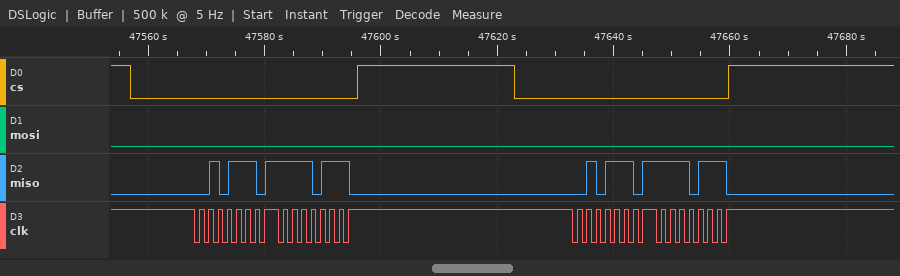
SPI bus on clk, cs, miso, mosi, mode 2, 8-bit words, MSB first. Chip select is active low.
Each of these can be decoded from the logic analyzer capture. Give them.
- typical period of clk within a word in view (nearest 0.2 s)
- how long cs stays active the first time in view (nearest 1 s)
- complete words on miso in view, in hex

1.6 s
39 s
2E, F7, 2E, F7
